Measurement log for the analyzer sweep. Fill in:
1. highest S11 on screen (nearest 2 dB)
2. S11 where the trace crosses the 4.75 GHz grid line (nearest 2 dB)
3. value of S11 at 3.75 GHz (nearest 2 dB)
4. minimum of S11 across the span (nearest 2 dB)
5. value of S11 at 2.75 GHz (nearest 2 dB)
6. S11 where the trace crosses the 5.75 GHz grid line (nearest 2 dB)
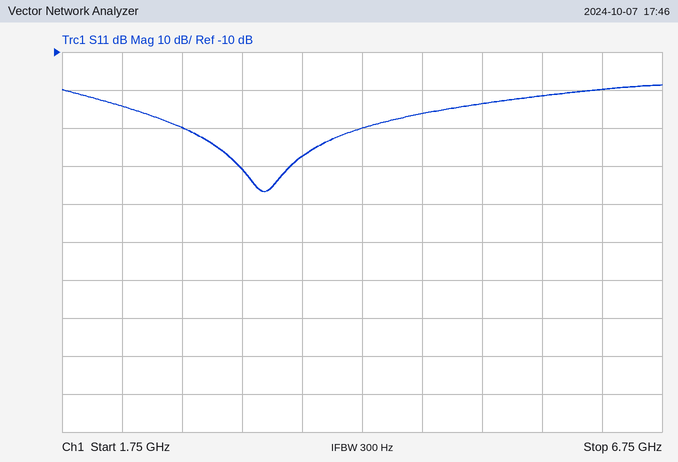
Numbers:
-18 dB
-26 dB
-38 dB
-46 dB
-30 dB
-22 dB
